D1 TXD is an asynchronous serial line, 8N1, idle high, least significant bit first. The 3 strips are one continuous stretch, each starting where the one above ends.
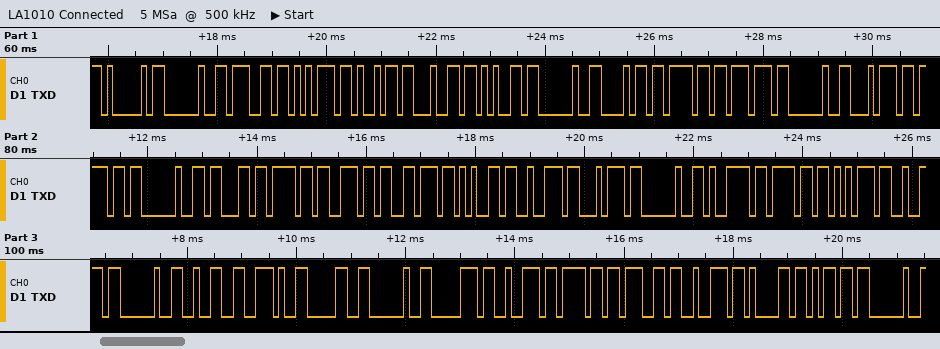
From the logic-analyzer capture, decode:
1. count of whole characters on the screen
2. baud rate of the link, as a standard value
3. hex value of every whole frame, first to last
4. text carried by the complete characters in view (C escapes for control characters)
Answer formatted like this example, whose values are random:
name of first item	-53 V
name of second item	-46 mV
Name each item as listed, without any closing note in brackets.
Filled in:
count of whole characters on the screen	40
baud rate of the link, as a standard value	9600 baud
hex value of every whole frame, first to last	41 20 67 75 69 64 65 20 68 6F 77 20 74 6F 20 63 6F 6E 76 65 72 74 20 79 6F 75 72 20 32 2E 30 20 70 72 6F 67 72 61 6D 20
text carried by the complete characters in view	"A guide how to convert your 2.0 program "
